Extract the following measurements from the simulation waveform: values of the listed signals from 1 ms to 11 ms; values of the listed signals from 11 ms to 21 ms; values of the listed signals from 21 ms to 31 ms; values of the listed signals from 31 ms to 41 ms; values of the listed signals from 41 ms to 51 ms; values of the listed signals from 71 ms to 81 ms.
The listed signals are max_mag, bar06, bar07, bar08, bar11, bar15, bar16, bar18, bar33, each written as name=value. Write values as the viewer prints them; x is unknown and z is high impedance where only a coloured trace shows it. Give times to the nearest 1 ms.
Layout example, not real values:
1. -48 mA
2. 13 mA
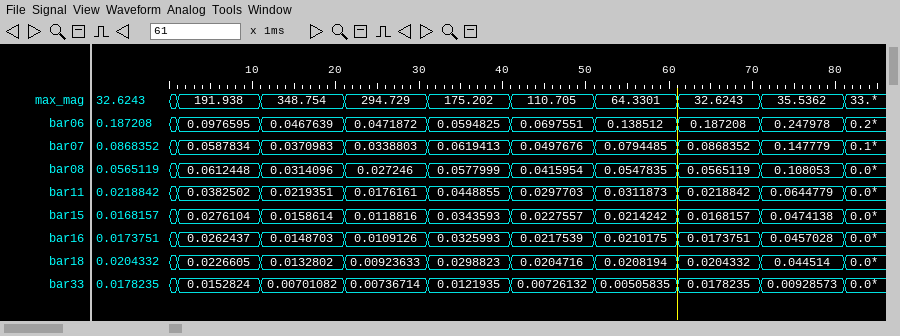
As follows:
1. max_mag=191.938, bar06=0.0976595, bar07=0.0587834, bar08=0.0612448, bar11=0.0382502, bar15=0.0276104, bar16=0.0262437, bar18=0.0226605, bar33=0.0152824
2. max_mag=348.754, bar06=0.0467639, bar07=0.0370983, bar08=0.0314096, bar11=0.0219351, bar15=0.0158614, bar16=0.0148703, bar18=0.0132802, bar33=0.00701082
3. max_mag=294.729, bar06=0.0471872, bar07=0.0338803, bar08=0.027246, bar11=0.0176161, bar15=0.0118816, bar16=0.0109126, bar18=0.00923633, bar33=0.00736714
4. max_mag=175.202, bar06=0.0594825, bar07=0.0619413, bar08=0.0577999, bar11=0.0448855, bar15=0.0343593, bar16=0.0325993, bar18=0.0298823, bar33=0.0121935
5. max_mag=110.705, bar06=0.0697551, bar07=0.0497676, bar08=0.0415954, bar11=0.0297703, bar15=0.0227557, bar16=0.0217539, bar18=0.0204716, bar33=0.00726132
6. max_mag=35.5362, bar06=0.247978, bar07=0.147779, bar08=0.108053, bar11=0.0644779, bar15=0.0474138, bar16=0.0457028, bar18=0.044514, bar33=0.00928573
